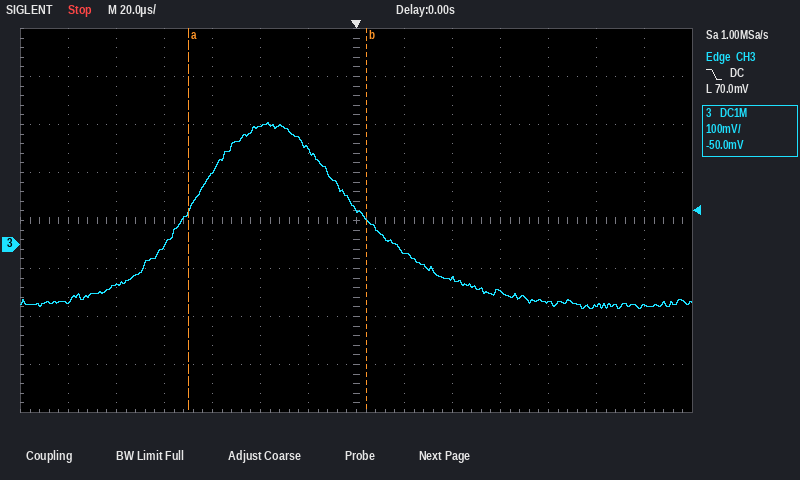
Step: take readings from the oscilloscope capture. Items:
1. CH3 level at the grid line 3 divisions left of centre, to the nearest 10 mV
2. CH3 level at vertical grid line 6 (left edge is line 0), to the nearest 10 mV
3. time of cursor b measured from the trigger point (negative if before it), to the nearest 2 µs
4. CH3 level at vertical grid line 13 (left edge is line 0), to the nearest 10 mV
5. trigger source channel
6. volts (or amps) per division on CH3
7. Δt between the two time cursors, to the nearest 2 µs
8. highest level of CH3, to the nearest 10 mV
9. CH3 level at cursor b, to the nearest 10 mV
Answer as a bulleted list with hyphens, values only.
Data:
- 150 mV
- 200 mV
- +4 µs
- -130 mV
- CH3
- 100 mV
- 74 µs
- 250 mV
- 50 mV
